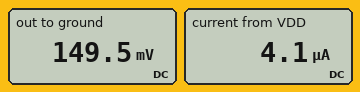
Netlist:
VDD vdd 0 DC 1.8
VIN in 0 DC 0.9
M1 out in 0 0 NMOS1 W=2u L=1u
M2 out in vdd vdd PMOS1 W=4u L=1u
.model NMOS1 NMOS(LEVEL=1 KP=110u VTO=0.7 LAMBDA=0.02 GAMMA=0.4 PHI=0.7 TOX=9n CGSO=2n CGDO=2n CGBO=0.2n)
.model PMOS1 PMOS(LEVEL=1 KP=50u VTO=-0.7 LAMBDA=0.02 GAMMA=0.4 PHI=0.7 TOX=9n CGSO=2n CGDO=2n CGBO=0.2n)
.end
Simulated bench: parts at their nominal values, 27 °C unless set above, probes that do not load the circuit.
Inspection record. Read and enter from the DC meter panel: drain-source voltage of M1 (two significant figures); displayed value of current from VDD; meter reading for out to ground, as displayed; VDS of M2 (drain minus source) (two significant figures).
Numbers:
150 mV
4.1 µA
149.5 mV
-1.7 V
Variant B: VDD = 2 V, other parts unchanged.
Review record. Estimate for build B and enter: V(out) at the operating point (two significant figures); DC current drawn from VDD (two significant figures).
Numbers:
1.9 V
4.6 µA
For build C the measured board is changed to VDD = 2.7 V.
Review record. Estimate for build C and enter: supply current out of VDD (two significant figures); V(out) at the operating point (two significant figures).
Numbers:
4.6 µA
2.7 V
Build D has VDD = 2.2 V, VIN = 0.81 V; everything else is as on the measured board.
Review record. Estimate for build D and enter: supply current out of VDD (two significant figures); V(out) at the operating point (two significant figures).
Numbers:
1.4 µA
2.2 V
